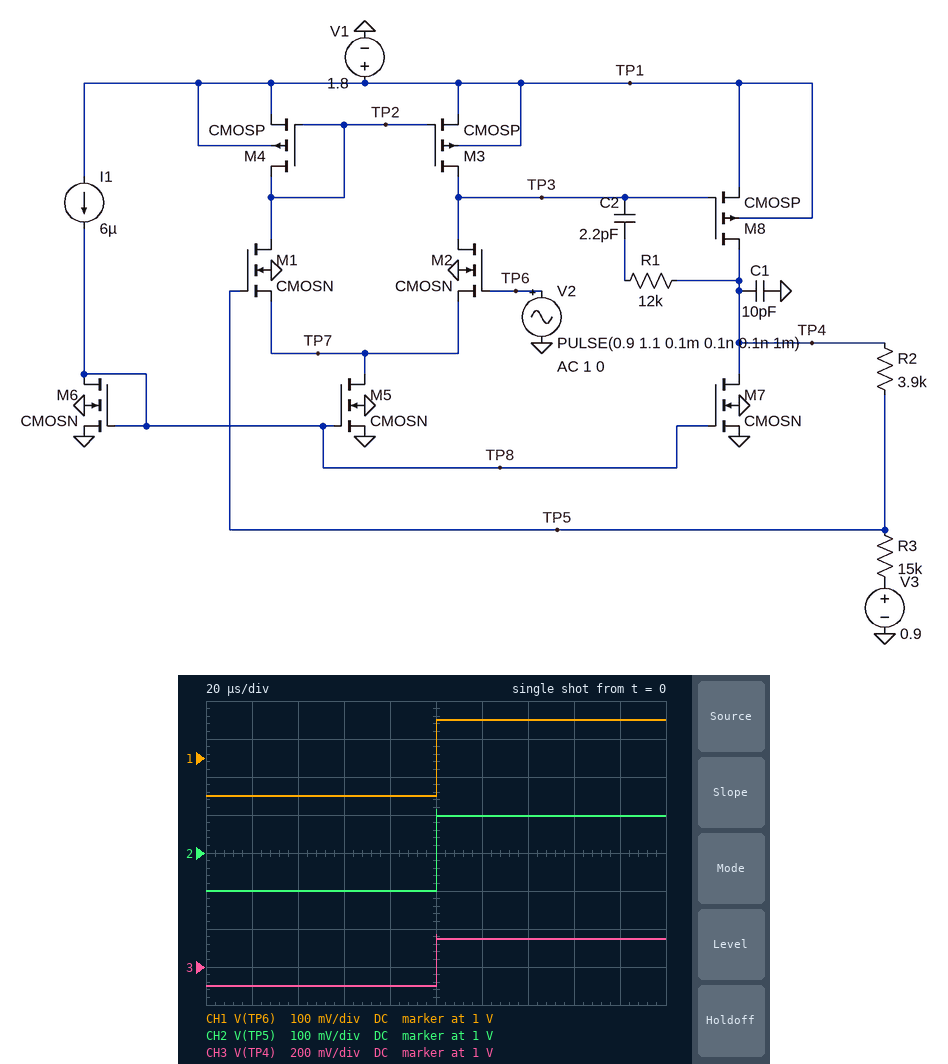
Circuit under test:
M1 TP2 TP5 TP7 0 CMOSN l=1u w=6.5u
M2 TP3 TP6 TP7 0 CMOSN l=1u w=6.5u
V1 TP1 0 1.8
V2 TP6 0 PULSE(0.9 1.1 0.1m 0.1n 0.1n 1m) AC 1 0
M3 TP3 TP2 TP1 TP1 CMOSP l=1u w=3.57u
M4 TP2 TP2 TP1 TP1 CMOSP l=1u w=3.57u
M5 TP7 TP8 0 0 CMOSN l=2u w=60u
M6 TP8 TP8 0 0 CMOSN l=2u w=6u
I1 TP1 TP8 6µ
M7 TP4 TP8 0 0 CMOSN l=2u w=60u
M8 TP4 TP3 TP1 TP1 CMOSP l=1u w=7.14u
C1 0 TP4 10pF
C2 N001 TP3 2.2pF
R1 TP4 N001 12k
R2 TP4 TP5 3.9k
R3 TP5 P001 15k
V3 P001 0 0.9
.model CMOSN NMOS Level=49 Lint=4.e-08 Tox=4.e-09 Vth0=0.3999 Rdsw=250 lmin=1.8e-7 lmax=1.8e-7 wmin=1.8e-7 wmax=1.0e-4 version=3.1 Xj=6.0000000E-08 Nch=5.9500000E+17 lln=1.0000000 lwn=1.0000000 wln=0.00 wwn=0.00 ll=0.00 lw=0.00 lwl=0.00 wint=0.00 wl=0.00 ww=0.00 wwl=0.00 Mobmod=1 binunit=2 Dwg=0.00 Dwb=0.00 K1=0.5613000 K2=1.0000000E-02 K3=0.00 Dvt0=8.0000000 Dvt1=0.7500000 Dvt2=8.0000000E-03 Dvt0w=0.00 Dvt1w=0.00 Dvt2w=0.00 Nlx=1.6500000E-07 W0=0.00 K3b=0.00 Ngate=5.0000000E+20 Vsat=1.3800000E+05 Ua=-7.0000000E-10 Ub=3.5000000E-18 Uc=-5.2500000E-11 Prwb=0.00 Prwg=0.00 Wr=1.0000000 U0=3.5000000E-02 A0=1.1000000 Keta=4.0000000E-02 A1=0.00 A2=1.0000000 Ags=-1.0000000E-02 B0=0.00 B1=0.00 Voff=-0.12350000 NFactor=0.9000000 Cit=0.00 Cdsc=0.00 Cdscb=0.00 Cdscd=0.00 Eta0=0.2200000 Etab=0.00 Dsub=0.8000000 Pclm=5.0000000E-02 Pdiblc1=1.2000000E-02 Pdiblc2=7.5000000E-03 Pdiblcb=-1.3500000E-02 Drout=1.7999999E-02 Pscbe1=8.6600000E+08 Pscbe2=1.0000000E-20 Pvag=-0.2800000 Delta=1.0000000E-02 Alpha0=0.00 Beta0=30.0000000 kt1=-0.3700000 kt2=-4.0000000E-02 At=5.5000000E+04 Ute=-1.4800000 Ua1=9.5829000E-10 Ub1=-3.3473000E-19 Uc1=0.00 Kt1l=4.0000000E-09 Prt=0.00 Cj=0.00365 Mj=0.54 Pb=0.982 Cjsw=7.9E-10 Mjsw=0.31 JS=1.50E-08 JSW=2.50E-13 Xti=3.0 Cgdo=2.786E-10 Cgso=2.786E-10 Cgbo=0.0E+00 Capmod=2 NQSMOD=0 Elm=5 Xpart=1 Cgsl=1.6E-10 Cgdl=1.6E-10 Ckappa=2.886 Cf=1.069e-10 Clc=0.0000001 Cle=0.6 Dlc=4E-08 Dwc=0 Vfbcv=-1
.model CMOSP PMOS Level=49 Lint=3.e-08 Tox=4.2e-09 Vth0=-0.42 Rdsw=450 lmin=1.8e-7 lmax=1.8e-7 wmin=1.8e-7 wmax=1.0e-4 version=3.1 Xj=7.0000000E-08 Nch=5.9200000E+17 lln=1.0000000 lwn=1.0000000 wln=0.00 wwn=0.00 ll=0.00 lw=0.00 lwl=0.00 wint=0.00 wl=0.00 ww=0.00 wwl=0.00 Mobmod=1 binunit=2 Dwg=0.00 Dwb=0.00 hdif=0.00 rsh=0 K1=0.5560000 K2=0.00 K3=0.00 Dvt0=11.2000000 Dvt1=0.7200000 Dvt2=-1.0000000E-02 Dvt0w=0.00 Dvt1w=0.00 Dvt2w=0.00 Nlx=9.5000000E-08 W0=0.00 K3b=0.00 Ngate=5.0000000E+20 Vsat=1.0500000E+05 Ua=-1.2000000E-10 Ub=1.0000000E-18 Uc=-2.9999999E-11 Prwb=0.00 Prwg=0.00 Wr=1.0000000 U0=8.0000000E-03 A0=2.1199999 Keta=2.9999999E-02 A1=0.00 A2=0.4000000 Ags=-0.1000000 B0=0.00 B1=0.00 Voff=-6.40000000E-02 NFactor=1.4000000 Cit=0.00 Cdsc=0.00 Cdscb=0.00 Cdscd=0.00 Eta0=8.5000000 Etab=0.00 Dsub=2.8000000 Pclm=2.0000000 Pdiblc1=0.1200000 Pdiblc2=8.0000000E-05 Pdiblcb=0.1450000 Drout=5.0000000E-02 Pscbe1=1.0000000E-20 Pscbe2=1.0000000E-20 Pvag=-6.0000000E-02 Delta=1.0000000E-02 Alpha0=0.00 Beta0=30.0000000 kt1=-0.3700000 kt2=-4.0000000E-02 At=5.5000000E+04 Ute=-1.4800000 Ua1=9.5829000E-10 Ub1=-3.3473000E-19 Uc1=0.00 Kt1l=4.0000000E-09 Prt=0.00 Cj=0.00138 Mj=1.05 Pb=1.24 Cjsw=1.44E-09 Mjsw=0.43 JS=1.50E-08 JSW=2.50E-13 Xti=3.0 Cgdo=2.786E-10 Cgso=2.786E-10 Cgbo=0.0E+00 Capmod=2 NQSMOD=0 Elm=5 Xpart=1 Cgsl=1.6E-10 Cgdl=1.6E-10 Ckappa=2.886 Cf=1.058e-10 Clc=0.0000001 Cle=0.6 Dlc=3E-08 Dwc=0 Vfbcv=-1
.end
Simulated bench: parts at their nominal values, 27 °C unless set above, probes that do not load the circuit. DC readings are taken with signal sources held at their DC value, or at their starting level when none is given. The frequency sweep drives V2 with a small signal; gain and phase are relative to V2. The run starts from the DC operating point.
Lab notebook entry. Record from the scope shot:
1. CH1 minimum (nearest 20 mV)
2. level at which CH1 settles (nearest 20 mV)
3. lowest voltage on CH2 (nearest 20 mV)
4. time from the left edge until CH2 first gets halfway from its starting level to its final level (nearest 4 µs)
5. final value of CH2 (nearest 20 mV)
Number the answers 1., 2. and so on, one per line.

1. 900 mV
2. 1.10 V
3. 900 mV
4. 100 µs
5. 1.10 V
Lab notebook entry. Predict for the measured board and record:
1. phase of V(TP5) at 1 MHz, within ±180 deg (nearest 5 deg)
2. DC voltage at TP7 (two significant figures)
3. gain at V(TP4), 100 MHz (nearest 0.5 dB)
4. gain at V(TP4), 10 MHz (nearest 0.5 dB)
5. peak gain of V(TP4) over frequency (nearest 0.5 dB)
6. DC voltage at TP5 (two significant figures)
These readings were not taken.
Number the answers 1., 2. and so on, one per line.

1. -5 deg
2. 220 mV
3. -29.5 dB
4. -3.5 dB
5. 3.0 dB
6. 900 mV
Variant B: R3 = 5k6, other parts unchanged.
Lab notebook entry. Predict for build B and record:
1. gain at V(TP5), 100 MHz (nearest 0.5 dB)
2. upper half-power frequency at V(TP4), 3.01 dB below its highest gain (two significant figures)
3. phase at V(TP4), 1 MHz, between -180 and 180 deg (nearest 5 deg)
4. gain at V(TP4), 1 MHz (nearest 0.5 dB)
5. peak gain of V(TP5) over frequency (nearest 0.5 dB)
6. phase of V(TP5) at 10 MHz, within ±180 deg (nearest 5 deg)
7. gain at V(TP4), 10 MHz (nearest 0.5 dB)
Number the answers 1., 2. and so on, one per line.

1. -35.5 dB
2. 6.1 MHz
3. -10 deg
4. 4.5 dB
5. 0 dB
6. -100 deg
7. -4.0 dB
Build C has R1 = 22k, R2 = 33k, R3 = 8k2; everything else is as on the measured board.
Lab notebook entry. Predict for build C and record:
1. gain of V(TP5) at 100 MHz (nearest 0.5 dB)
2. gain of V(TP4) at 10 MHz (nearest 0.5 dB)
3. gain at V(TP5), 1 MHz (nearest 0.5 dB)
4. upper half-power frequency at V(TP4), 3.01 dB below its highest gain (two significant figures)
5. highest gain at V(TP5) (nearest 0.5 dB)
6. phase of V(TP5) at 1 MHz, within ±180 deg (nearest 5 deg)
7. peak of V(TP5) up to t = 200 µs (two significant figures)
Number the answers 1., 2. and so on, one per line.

1. -23.0 dB
2. 0.5 dB
3. -0.5 dB
4. 2.9 MHz
5. 0 dB
6. -20 deg
7. 1.0 V
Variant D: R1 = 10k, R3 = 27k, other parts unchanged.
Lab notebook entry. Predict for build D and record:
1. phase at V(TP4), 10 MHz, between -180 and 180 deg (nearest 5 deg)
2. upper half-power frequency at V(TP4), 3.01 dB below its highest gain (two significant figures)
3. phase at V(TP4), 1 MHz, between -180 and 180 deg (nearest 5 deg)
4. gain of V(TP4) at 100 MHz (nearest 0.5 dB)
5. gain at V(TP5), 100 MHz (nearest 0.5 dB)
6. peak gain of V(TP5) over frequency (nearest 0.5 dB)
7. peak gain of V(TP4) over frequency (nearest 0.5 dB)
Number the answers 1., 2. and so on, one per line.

1. -110 deg
2. 7.8 MHz
3. -5 deg
4. -32.5 dB
5. -31.0 dB
6. 2.0 dB
7. 3.5 dB
